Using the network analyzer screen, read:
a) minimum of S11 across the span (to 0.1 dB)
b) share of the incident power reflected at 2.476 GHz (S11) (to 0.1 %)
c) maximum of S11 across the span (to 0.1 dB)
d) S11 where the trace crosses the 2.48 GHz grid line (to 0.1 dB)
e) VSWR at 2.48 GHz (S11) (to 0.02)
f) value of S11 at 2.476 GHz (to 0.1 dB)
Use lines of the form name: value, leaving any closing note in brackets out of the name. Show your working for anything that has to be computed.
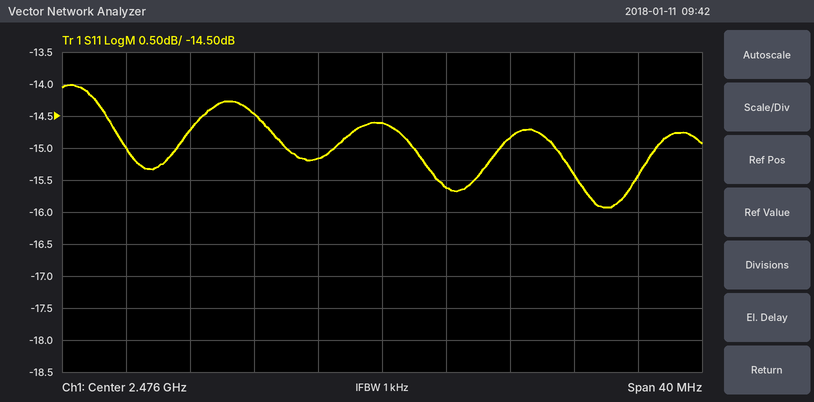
minimum of S11 across the span: -15.9 dB
share of the incident power reflected at 2.476 GHz (S11): 10^(-14.6/10) ≈ 3.5 %
maximum of S11 across the span: -14.0 dB
S11 where the trace crosses the 2.48 GHz grid line: -15.6 dB
VSWR at 2.48 GHz (S11): |Γ| = 10^(-15.6/20) = 0.1660; VSWR = (1 + 0.1660)/(1 − 0.1660) ≈ 1.40
value of S11 at 2.476 GHz: -14.6 dB
